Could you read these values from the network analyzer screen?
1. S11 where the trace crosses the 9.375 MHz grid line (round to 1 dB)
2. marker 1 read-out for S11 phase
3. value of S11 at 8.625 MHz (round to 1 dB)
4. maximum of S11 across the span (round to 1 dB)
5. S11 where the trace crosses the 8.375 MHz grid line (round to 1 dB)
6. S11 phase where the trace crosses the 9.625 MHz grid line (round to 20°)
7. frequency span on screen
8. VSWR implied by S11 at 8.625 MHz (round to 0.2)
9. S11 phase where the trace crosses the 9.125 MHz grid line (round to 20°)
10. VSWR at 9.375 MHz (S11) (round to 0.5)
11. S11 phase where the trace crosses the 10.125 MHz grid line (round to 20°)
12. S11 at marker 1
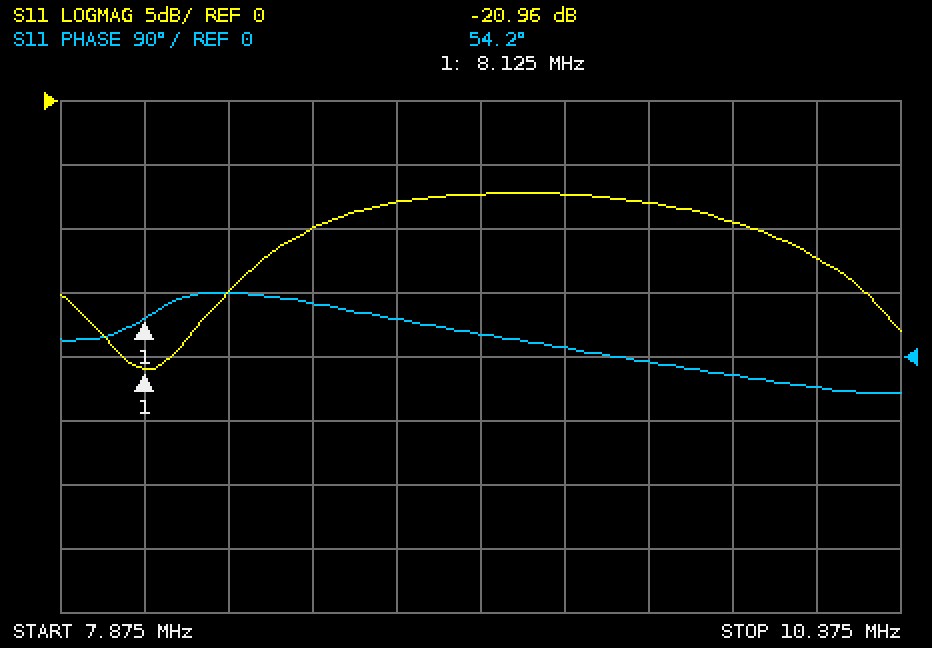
-7 dB
54.2°
-10 dB
-7 dB
-15 dB
0°
2.5 MHz
2.0
40°
2.5
-40°
-20.96 dB
